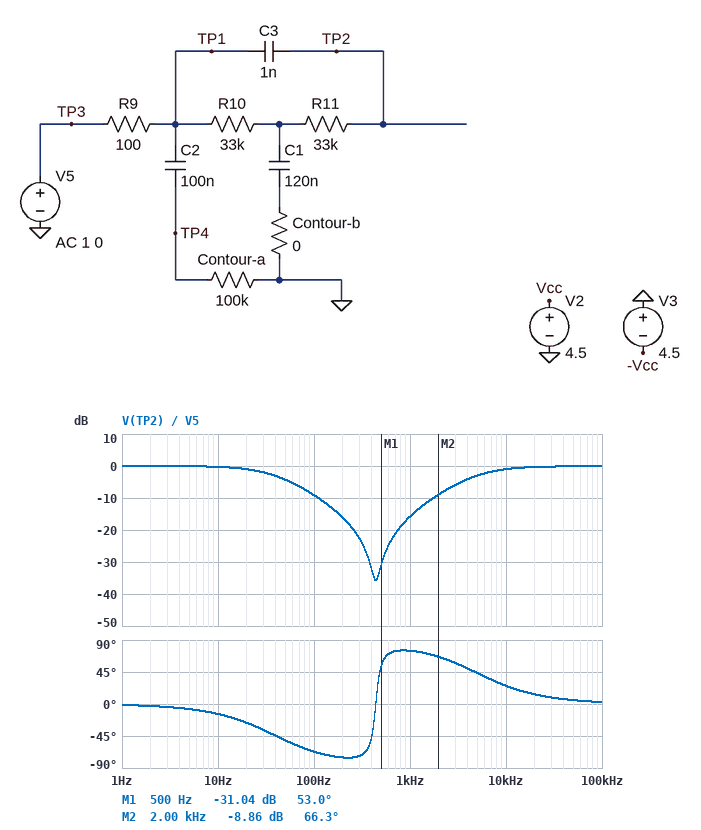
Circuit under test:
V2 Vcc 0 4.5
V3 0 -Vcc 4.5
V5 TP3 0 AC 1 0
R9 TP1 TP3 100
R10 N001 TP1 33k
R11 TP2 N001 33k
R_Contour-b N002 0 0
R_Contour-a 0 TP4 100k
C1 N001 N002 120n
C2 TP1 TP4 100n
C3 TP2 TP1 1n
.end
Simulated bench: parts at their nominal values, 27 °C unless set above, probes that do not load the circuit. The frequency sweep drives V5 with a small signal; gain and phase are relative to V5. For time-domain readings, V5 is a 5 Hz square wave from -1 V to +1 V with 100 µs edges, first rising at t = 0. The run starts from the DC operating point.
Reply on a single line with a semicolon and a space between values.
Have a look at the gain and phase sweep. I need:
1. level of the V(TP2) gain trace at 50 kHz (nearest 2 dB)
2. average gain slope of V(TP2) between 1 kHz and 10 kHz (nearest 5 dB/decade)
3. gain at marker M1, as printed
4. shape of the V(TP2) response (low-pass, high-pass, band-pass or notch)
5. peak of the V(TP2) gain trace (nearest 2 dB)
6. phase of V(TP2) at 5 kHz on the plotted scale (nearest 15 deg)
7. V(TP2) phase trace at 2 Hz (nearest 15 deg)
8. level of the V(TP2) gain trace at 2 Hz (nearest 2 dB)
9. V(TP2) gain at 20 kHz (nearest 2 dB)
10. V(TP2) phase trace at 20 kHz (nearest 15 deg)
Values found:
0 dB; 15 dB/decade; -31.04 dB; notch; 0 dB; 45 deg; 0 deg; 0 dB; 0 dB; 15 deg
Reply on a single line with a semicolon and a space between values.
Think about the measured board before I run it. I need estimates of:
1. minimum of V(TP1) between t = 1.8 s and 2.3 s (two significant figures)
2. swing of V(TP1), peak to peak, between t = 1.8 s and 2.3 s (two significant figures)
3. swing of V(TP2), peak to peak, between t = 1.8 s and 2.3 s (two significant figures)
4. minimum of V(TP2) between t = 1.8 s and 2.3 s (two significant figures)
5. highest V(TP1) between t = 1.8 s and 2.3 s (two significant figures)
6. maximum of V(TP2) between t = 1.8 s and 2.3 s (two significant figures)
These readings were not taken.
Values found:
-1.0 V; 2.0 V; 2.0 V; -1.0 V; 1.0 V; 1.0 V
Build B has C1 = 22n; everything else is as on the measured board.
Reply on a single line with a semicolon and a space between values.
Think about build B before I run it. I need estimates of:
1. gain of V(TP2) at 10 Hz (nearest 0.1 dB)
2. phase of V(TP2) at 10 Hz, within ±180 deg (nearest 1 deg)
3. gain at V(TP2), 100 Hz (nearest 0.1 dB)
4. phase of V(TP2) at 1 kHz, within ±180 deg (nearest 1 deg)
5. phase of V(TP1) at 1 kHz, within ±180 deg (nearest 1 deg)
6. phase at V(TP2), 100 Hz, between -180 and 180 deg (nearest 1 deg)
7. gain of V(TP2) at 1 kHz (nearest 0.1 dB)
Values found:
0 dB; -3 deg; -1.0 dB; -7 deg; 0 deg; -24 deg; -21.5 dB
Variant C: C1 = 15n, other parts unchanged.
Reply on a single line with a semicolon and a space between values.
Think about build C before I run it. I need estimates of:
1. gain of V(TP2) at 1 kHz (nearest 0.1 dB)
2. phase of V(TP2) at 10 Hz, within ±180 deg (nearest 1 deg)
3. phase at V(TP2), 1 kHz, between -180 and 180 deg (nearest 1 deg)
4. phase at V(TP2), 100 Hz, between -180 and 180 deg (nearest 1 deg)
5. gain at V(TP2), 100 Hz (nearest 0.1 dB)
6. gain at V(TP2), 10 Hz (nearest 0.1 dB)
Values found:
-16.3 dB; -2 deg; -35 deg; -17 deg; -0.5 dB; 0 dB
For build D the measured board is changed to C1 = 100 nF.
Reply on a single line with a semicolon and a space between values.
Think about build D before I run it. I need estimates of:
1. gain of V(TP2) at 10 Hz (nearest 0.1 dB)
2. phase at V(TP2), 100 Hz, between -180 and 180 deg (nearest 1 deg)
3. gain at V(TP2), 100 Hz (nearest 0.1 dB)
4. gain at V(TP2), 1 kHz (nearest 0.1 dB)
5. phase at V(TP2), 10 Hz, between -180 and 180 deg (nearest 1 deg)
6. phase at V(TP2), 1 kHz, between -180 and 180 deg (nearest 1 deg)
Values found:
-0.2 dB; -63 deg; -7.7 dB; -16.2 dB; -12 deg; 74 deg
